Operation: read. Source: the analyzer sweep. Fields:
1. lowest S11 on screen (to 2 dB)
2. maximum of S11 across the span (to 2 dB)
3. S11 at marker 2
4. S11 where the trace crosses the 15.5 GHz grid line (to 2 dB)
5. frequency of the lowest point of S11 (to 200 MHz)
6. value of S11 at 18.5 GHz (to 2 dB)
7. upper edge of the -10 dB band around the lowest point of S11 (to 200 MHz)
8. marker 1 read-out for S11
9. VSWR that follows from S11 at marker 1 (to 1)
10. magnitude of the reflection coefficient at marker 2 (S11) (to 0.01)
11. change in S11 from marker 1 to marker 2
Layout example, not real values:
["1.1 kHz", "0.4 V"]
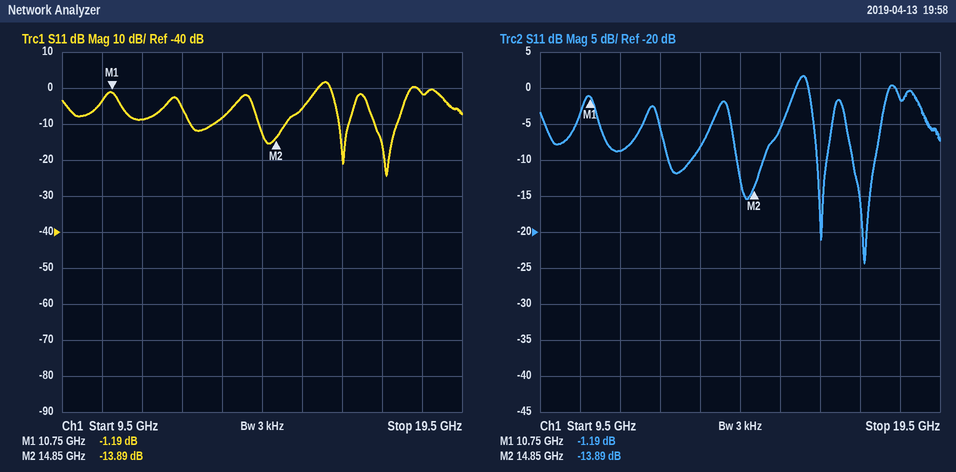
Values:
["-24 dB", "2 dB", "-13.89 dB", "-6 dB", "17.6 GHz", "-2 dB", "17.8 GHz", "-1.19 dB", "15", "0.20", "-12.70 dB"]
